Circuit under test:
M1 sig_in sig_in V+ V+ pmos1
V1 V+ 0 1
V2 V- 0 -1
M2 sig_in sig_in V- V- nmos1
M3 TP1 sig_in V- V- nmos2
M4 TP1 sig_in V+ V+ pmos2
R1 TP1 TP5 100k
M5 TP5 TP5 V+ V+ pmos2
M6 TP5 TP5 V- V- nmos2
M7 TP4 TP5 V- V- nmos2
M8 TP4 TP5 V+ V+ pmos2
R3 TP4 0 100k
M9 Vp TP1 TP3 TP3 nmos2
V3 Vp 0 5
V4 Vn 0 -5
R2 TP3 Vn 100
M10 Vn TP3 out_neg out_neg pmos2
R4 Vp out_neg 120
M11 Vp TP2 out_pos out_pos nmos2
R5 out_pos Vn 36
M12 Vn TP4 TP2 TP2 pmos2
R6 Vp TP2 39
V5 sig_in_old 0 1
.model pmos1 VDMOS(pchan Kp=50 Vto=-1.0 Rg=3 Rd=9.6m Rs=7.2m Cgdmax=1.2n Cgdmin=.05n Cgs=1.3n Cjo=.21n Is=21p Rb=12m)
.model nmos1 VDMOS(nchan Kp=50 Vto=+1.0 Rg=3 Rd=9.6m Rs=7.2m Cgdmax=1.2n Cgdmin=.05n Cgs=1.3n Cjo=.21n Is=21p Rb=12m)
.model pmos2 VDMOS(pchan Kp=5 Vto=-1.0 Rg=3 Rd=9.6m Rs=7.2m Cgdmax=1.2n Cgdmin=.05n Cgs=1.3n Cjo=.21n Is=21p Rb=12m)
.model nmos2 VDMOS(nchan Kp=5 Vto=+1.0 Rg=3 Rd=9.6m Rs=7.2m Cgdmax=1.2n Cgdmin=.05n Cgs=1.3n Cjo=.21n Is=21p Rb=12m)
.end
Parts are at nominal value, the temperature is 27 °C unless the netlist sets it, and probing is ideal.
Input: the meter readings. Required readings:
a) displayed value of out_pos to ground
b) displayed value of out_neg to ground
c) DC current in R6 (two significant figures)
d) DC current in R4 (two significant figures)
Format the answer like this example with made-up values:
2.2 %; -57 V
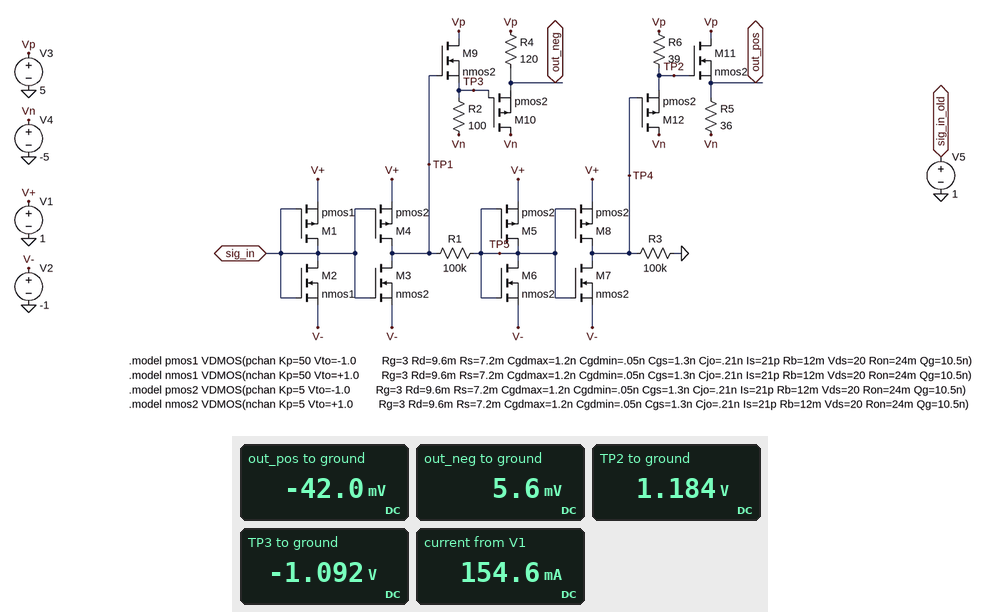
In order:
-42.0 mV; 5.6 mV; 98 mA; 42 mA
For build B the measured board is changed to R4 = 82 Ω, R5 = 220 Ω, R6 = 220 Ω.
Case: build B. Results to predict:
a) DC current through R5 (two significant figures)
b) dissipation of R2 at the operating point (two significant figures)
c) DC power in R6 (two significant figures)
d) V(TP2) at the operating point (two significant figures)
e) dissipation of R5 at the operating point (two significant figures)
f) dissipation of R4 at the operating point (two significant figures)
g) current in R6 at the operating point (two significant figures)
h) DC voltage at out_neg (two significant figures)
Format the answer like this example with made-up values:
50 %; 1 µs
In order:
23 mA; 150 mW; 72 mW; 1.0 V; 110 mW; 300 mW; 18 mA; 41 mV
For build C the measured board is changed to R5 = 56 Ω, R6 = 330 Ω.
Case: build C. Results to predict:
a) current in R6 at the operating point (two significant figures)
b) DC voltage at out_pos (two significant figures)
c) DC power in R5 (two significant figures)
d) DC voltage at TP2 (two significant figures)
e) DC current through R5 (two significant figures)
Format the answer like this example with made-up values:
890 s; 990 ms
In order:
12 mA; -170 mV; 420 mW; 1.0 V; 86 mA
